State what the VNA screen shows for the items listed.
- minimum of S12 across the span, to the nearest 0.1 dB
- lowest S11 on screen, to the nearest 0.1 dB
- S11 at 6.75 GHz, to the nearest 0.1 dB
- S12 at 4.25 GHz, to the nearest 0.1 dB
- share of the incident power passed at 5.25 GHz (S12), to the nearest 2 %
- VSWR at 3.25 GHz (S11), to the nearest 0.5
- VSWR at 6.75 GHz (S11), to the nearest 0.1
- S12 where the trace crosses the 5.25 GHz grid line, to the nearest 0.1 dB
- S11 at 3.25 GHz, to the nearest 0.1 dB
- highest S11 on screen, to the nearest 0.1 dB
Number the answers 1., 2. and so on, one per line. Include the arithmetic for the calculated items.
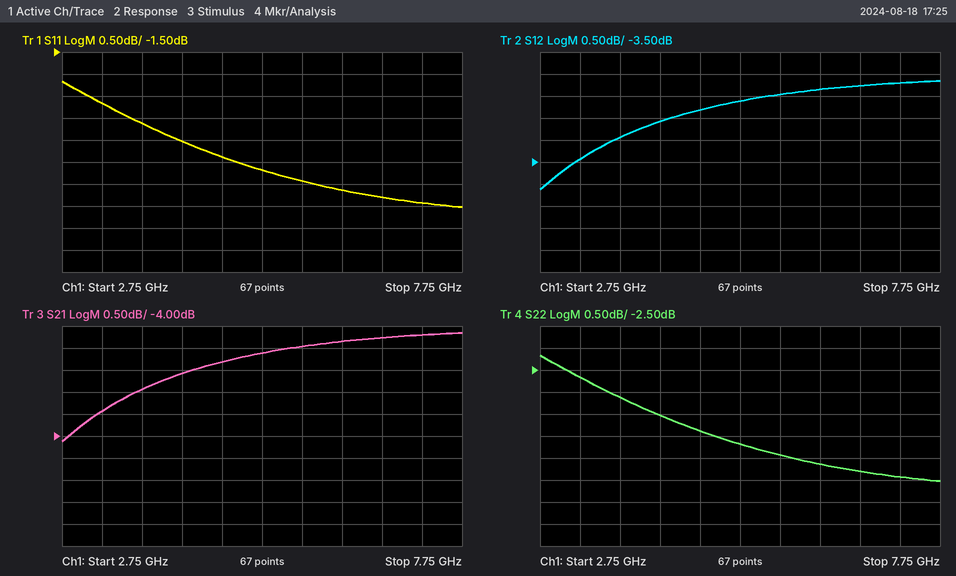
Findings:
1. -4.1 dB
2. -5.0 dB
3. -4.8 dB
4. -2.6 dB
5. 10^(-2.1/10) ≈ 62 %
6. |Γ| = 10^(-2.7/20) = 0.7328; VSWR = (1 + 0.7328)/(1 − 0.7328) ≈ 6.5
7. |Γ| = 10^(-4.8/20) = 0.5754; VSWR = (1 + 0.5754)/(1 − 0.5754) ≈ 3.7
8. -2.1 dB
9. -2.7 dB
10. -2.2 dB
